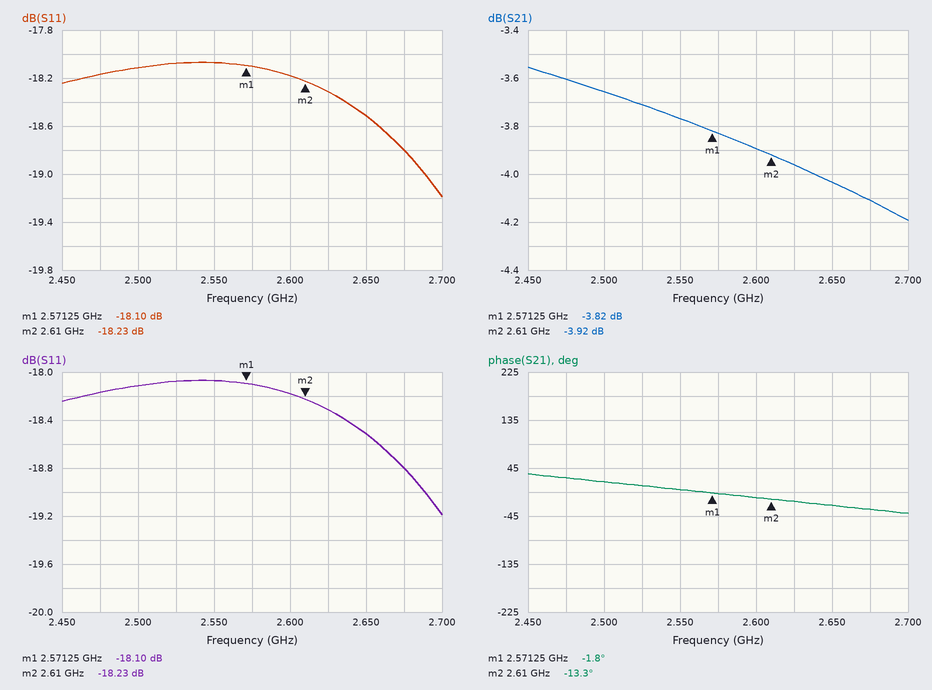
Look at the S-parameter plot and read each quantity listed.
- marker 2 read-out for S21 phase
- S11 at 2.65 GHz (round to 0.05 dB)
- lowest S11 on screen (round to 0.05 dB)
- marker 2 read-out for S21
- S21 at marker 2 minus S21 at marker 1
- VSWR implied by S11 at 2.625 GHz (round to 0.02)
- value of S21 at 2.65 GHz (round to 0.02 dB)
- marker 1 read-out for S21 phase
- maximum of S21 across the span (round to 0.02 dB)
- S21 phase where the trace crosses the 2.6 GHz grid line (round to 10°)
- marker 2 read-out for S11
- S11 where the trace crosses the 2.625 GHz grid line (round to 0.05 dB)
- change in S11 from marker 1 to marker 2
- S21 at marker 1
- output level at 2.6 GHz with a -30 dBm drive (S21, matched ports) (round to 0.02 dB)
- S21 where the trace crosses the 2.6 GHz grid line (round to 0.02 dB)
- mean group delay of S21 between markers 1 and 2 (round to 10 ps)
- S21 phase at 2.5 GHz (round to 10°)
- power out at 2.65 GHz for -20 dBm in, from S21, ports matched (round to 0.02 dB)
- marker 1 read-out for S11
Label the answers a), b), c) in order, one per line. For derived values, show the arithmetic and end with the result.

a) -13.3°
b) -18.50 dB
c) -19.20 dB
d) -3.92 dB
e) -3.92 − (-3.82) = -0.10 dB
f) |Γ| = 10^(-18.3/20) = 0.1216; VSWR = (1 + 0.1216)/(1 − 0.1216) ≈ 1.28
g) -4.04 dB
h) -1.8°
i) -3.56 dB
j) -10°
k) -18.23 dB
l) -18.30 dB
m) -18.23 − (-18.1) = -0.13 dB
n) -3.82 dB
o) -30 dBm + (-3.90 dB) = -33.90 dBm
p) -3.90 dB
q) −(-13.3° − (-1.8°))/(360° × 38.75 MHz) ≈ 824 ps, so 820 ps to the nearest 10 ps
r) 20°
s) -20 dBm + (-4.04 dB) = -24.04 dBm
t) -18.10 dB
